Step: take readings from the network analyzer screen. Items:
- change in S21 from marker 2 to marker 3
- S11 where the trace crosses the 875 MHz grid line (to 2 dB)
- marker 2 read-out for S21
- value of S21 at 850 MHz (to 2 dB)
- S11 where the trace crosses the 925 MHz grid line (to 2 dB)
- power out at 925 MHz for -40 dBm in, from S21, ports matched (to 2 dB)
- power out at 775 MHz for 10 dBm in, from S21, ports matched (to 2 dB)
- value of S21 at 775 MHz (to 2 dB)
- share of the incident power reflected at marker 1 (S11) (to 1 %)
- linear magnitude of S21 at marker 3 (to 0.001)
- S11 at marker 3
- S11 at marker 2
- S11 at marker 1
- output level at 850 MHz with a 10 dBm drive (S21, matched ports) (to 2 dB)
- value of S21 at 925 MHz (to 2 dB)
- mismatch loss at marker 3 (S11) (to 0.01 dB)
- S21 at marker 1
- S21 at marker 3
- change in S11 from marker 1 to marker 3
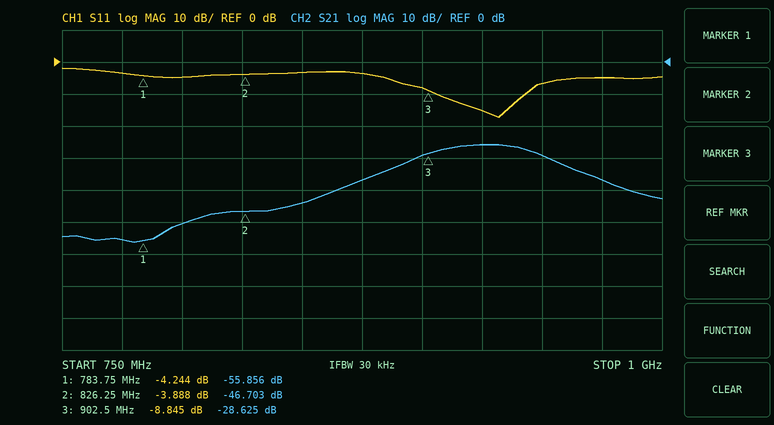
18.078 dB
-4 dB
-46.703 dB
-44 dB
-16 dB
-66 dBm
-46 dBm
-56 dB
38 %
0.037
-8.845 dB
-3.888 dB
-4.244 dB
-34 dBm
-26 dB
0.61 dB
-55.856 dB
-28.625 dB
-4.601 dB
